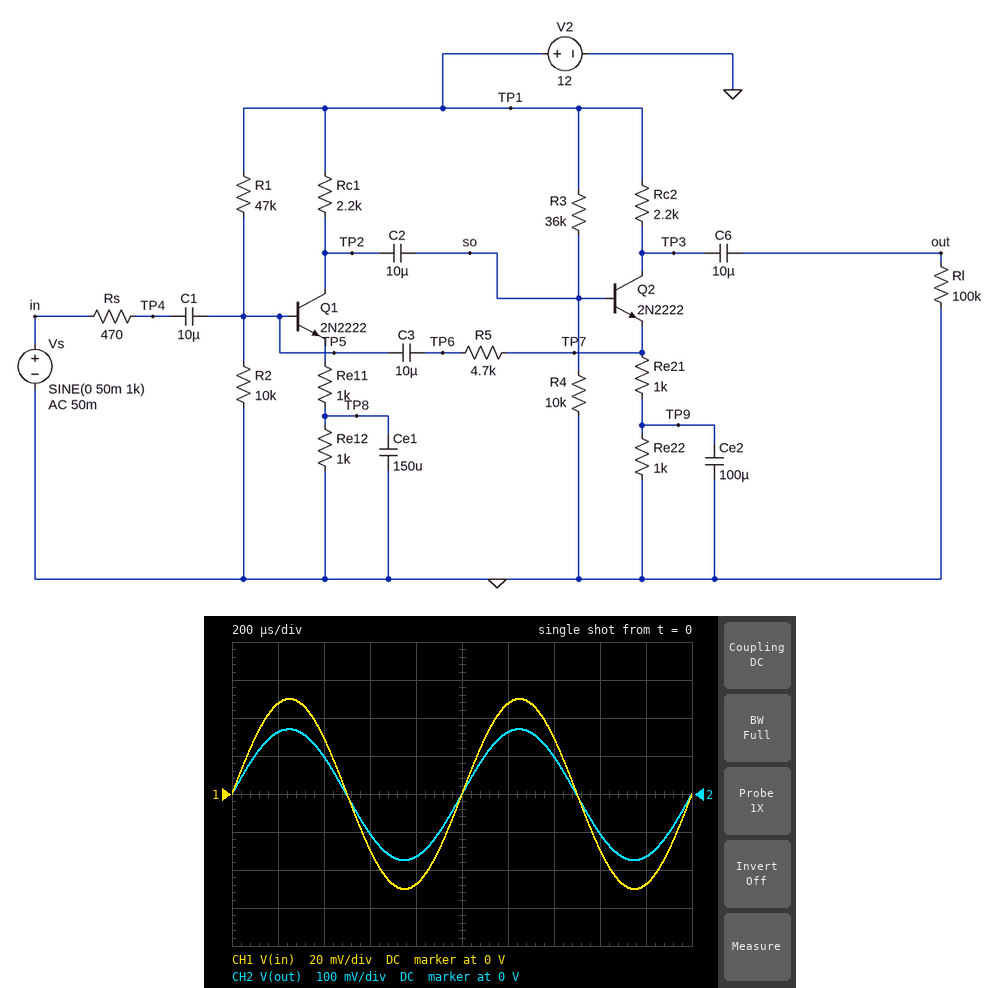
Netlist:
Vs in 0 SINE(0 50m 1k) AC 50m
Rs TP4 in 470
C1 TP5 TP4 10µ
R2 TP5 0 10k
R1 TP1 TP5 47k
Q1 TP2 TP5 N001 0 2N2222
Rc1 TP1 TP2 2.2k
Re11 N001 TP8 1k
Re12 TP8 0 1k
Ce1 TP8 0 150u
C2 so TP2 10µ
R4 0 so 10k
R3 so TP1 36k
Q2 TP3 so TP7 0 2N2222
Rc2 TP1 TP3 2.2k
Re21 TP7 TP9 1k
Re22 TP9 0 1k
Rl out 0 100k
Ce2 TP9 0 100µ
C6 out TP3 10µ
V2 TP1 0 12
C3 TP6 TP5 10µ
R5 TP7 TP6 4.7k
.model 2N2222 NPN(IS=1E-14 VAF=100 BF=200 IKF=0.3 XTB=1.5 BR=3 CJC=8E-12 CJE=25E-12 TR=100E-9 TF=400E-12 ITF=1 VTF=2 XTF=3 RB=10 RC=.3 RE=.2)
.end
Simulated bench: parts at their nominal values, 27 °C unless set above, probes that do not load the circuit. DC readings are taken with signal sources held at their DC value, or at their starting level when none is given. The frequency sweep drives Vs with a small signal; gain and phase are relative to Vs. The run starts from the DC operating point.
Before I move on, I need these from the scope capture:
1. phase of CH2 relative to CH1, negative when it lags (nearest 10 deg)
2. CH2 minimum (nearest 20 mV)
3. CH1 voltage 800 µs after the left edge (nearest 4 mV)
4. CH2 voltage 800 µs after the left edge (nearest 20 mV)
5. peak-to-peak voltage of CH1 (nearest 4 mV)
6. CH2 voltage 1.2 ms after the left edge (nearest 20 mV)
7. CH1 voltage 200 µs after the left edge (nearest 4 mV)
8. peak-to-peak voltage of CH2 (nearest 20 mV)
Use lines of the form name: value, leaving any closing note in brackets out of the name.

phase of CH2 relative to CH1, negative when it lags: 0 deg
CH2 minimum: -180 mV
CH1 voltage 800 µs after the left edge: -48 mV
CH2 voltage 800 µs after the left edge: -160 mV
peak-to-peak voltage of CH1: 100 mV
CH2 voltage 1.2 ms after the left edge: 160 mV
CH1 voltage 200 µs after the left edge: 48 mV
peak-to-peak voltage of CH2: 340 mV
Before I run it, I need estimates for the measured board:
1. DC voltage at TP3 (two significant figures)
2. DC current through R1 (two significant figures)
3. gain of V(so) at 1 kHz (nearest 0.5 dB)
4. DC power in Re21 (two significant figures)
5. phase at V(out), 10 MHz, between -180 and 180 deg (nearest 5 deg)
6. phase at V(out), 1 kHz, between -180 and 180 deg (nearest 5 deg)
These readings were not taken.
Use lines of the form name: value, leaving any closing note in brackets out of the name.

DC voltage at TP3: 9.9 V
DC current through R1: 210 µA
gain of V(so) at 1 kHz: 2.0 dB
DC power in Re21: 920 µW
phase at V(out), 10 MHz, between -180 and 180 deg: -105 deg
phase at V(out), 1 kHz, between -180 and 180 deg: 0 deg
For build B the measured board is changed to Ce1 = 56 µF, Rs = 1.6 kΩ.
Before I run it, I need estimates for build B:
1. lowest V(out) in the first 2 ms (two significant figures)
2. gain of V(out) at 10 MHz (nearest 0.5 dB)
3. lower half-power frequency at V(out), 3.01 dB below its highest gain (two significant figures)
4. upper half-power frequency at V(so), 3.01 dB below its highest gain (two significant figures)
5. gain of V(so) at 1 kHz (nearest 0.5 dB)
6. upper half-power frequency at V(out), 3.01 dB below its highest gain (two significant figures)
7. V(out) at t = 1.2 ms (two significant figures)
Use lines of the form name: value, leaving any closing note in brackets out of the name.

lowest V(out) in the first 2 ms: -110 mV
gain of V(out) at 10 MHz: -0.5 dB
lower half-power frequency at V(out), 3.01 dB below its highest gain: 7.9 Hz
upper half-power frequency at V(so), 3.01 dB below its highest gain: 5.3 MHz
gain of V(so) at 1 kHz: -2.0 dB
upper half-power frequency at V(out), 3.01 dB below its highest gain: 4.9 MHz
V(out) at t = 1.2 ms: 100 mV
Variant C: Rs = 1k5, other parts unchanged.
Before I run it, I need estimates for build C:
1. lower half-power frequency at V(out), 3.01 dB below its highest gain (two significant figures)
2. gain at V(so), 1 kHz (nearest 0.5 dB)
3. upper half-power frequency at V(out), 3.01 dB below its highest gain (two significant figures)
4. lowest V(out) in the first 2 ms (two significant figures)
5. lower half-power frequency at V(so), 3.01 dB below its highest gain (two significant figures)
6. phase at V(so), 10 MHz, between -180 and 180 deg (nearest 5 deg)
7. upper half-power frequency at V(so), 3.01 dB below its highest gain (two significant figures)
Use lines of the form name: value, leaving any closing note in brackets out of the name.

lower half-power frequency at V(out), 3.01 dB below its highest gain: 7.1 Hz
gain at V(so), 1 kHz: -2.0 dB
upper half-power frequency at V(out), 3.01 dB below its highest gain: 4.9 MHz
lowest V(out) in the first 2 ms: -110 mV
lower half-power frequency at V(so), 3.01 dB below its highest gain: 5.8 Hz
phase at V(so), 10 MHz, between -180 and 180 deg: 100 deg
upper half-power frequency at V(so), 3.01 dB below its highest gain: 5.2 MHz
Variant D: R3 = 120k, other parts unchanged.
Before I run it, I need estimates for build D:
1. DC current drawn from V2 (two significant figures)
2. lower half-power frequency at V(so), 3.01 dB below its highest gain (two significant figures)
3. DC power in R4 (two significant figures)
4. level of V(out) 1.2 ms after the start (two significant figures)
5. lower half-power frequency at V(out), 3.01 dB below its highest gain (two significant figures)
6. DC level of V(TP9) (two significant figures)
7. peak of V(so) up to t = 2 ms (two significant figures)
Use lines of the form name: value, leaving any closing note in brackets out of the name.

DC current drawn from V2: 1.2 mA
lower half-power frequency at V(so), 3.01 dB below its highest gain: 9.8 Hz
DC power in R4: 84 µW
level of V(out) 1.2 ms after the start: 140 mV
lower half-power frequency at V(out), 3.01 dB below its highest gain: 10 Hz
DC level of V(TP9): 160 mV
peak of V(so) up to t = 2 ms: 980 mV
